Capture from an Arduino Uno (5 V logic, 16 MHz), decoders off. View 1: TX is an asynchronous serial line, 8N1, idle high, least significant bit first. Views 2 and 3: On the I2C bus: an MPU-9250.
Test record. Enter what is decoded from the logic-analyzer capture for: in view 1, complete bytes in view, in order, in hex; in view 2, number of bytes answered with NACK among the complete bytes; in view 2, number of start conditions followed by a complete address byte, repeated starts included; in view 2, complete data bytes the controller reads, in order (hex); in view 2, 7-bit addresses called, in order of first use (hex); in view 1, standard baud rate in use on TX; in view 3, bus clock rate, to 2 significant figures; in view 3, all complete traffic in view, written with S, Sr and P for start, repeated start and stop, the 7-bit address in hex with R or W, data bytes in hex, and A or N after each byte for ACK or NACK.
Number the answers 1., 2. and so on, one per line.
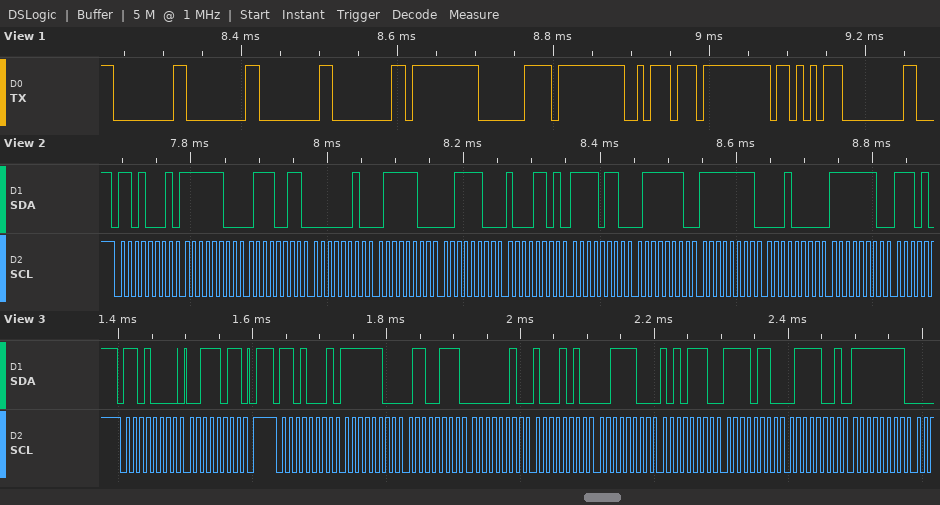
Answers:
1. 00 00 00 00 FF C0 FF BA FF AB 00
2. 0
3. 1
4. FC 73 02 7C 3C 8D F6 7E FF 10 FE
5. 0x68
6. 115200 baud
7. 100 kHz
8. S 68W A 3B A P S 68R A FC A 67 A 02 A 8A A 3C A AE A F6 A 79 A FF A
